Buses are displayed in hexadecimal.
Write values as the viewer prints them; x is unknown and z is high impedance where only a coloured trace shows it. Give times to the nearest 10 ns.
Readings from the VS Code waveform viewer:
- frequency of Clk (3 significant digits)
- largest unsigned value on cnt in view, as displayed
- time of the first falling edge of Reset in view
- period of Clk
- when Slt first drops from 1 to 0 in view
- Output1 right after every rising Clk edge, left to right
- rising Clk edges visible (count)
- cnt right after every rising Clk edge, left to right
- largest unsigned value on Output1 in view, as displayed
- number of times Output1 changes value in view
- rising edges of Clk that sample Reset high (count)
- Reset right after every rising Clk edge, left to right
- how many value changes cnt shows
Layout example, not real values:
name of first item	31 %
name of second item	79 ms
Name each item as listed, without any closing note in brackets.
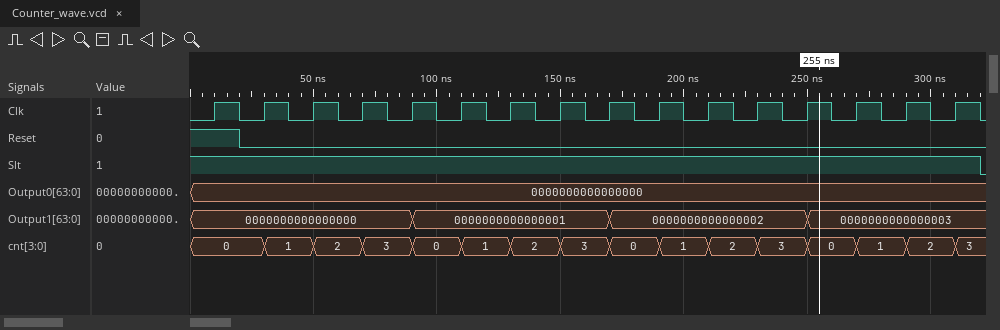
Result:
frequency of Clk	50.0 MHz
largest unsigned value on cnt in view, as displayed	3
time of the first falling edge of Reset in view	20 ns
period of Clk	20 ns
when Slt first drops from 1 to 0 in view	320 ns
Output1 right after every rising Clk edge, left to right	0000000000000000, 0000000000000000, 0000000000000000, 0000000000000000, 0000000000000001, 0000000000000001, 0000000000000001, 0000000000000001, 0000000000000002, 0000000000000002, 0000000000000002, 0000000000000002, 0000000000000003, 0000000000000003, 0000000000000003, 0000000000000003
rising Clk edges visible	16
cnt right after every rising Clk edge, left to right	0, 1, 2, 3, 0, 1, 2, 3, 0, 1, 2, 3, 0, 1, 2, 3
largest unsigned value on Output1 in view, as displayed	0000000000000003
number of times Output1 changes value in view	3
rising edges of Clk that sample Reset high	1
Reset right after every rising Clk edge, left to right	1 0 0 0 0 0 0 0 0 0 0 0 0 0 0 0
how many value changes cnt shows	15
